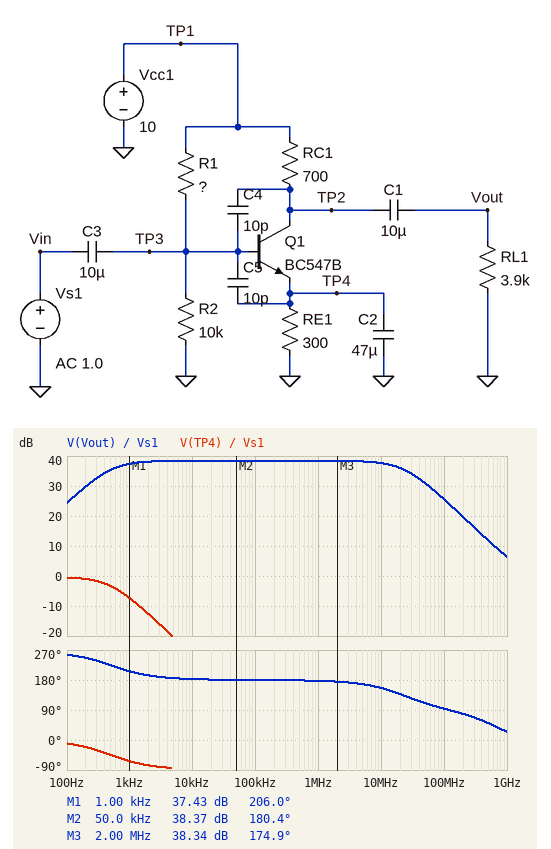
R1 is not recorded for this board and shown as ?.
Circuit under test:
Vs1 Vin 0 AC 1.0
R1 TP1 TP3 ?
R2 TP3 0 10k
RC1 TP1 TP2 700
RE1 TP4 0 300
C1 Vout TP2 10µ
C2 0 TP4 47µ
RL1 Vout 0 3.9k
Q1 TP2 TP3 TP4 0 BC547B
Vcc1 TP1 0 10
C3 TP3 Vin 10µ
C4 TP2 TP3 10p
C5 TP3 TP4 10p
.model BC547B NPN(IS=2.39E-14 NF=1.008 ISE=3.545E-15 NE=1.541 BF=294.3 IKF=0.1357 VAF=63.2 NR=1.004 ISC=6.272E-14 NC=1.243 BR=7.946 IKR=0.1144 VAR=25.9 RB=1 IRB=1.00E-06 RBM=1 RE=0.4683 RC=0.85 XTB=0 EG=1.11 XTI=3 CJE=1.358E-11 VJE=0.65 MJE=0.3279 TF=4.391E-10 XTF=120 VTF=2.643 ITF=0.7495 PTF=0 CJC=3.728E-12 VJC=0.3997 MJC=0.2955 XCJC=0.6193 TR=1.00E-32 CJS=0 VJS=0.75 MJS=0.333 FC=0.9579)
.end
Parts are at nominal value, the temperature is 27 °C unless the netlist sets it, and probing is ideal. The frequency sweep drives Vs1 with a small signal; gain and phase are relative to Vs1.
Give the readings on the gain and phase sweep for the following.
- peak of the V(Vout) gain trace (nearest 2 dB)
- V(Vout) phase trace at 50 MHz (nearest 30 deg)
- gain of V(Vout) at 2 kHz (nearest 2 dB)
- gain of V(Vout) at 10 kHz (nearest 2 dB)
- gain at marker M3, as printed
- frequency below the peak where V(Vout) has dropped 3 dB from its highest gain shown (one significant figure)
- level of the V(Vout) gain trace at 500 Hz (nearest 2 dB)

38 dB
120 deg
38 dB
38 dB
38.34 dB
500 Hz
36 dB
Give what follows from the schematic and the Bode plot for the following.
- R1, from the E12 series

39 kΩ
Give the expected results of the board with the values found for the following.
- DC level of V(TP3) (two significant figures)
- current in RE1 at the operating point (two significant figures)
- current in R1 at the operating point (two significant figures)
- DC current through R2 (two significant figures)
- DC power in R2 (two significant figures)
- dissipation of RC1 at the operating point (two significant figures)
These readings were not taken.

1.9 V
4.2 mA
210 µA
190 µA
370 µW
12 mW
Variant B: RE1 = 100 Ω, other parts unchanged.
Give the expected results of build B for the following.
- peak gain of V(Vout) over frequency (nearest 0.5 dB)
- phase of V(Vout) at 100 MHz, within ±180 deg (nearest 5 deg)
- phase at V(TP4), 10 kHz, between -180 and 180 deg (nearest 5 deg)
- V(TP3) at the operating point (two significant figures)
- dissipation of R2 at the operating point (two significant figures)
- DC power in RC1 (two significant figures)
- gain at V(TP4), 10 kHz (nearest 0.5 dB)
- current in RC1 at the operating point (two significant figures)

44.5 dB
90 deg
-85 deg
1.7 V
300 µW
74 mW
-20.0 dB
10 mA
